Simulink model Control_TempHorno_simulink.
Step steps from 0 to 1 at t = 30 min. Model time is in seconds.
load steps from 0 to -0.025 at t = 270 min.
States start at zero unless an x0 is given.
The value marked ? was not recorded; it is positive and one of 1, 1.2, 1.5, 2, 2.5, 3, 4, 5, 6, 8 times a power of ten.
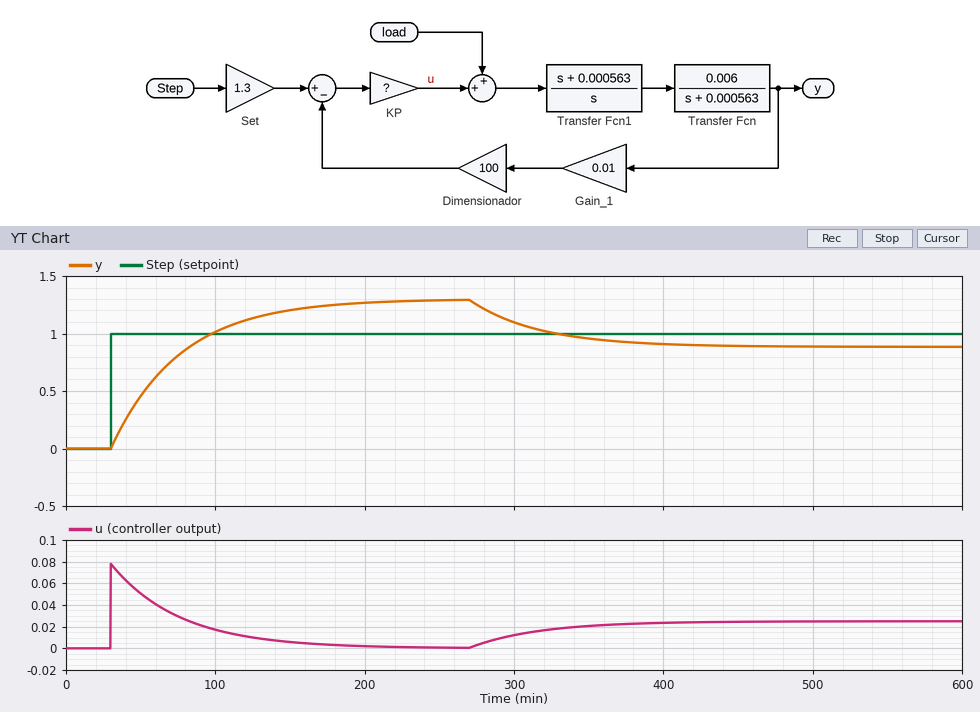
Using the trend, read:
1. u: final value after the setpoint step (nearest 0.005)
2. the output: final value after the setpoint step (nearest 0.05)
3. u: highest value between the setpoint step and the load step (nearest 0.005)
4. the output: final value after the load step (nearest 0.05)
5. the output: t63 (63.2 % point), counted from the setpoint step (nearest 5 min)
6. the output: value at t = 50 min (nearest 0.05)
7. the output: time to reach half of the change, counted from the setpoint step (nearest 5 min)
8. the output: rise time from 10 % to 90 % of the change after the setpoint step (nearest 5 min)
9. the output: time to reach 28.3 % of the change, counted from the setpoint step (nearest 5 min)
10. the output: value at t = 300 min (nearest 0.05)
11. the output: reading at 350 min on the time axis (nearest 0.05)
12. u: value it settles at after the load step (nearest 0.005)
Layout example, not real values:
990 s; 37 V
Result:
0.000; 1.30; 0.080; 0.90; 45 min; 0.45; 30 min; 100 min; 15 min; 1.10; 0.95; 0.025
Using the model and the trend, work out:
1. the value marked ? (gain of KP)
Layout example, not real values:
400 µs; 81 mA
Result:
0.06
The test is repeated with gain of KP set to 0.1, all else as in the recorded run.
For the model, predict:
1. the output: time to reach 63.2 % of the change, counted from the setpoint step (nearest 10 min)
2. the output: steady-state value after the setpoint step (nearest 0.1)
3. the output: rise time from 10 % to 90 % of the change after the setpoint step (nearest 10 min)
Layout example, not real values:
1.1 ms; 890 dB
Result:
30 min; 1.3; 60 min
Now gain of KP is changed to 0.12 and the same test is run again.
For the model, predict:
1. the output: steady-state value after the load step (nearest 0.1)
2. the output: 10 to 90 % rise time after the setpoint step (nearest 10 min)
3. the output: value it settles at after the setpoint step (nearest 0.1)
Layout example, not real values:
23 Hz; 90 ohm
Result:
1.1; 50 min; 1.3
